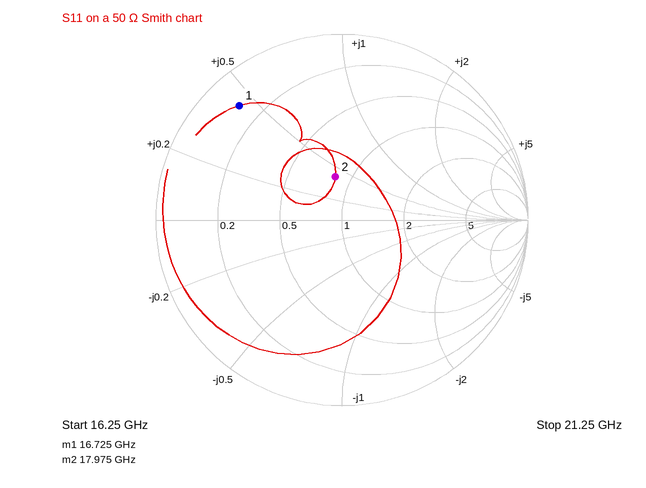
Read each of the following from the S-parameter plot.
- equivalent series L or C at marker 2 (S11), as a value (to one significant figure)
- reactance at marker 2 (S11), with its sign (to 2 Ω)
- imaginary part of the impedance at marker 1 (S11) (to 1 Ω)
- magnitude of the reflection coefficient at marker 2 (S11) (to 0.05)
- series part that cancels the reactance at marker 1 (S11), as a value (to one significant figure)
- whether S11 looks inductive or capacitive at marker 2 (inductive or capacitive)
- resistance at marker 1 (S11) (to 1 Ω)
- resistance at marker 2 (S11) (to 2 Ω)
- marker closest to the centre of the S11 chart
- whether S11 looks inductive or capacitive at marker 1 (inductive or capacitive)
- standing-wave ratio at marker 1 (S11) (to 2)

200 pH
+20 Ω
+22 Ω
0.25
400 fF
inductive
6 Ω
42 Ω
marker 2
inductive
10
